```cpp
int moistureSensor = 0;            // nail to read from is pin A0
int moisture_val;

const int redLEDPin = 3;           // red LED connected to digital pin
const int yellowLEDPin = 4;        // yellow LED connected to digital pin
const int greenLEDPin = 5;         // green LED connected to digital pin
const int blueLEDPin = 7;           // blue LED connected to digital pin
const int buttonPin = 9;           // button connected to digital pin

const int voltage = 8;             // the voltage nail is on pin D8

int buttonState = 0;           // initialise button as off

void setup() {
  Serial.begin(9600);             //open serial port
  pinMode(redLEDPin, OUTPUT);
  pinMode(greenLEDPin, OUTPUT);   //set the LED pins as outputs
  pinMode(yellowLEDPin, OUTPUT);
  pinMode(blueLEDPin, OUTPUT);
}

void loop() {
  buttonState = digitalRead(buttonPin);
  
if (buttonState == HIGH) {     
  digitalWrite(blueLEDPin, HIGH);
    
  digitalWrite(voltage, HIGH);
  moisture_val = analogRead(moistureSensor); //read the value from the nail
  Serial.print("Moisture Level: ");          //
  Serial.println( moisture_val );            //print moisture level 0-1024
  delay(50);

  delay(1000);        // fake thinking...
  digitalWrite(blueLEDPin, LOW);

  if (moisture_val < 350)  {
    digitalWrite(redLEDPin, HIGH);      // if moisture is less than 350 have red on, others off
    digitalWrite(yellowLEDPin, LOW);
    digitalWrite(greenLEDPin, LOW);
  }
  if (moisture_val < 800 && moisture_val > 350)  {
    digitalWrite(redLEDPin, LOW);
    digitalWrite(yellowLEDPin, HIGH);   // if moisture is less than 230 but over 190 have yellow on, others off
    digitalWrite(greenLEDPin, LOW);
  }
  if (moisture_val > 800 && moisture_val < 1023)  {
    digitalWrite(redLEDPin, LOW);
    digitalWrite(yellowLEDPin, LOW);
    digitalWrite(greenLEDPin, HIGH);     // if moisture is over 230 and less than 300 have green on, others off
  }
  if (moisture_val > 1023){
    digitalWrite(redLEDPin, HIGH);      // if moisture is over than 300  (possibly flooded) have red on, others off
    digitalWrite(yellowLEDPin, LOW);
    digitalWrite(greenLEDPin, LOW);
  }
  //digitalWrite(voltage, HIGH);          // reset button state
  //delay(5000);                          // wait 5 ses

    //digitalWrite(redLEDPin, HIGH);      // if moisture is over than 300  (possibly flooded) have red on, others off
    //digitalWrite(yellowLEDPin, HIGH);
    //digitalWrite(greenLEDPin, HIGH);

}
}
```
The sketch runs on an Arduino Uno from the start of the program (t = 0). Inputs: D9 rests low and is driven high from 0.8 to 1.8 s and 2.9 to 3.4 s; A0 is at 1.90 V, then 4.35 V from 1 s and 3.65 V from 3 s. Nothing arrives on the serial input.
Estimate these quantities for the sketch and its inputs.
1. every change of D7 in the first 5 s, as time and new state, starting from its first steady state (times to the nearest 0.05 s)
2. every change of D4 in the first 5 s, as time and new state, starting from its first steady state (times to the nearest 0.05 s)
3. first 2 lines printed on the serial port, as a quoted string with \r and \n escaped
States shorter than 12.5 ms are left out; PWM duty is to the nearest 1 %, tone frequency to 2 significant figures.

0 s low; 0.8 s high; 1.85 s low; 2.9 s high; 3.95 s low
0 s low; 1.85 s high; 3.95 s low
"Moisture Level: 389\r\nMoisture Level: 890\r\n"
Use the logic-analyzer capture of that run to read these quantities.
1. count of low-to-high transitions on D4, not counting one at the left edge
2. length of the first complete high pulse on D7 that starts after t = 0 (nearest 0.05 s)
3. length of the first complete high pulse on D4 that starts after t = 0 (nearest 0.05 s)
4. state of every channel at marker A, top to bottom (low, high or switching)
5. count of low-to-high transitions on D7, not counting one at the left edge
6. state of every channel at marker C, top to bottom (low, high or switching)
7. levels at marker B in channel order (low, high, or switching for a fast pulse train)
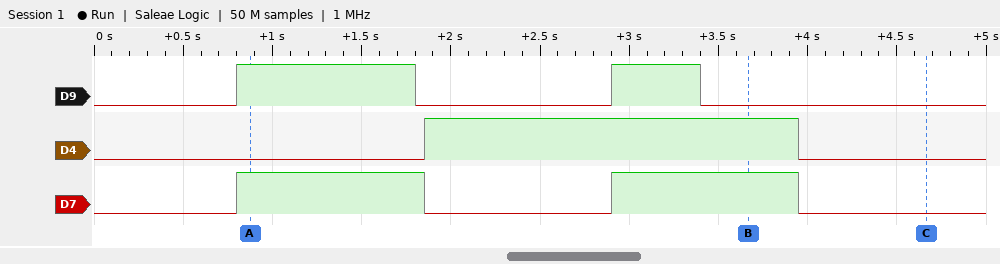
1
1.05 s
2.10 s
D9 high, D4 low, D7 high
2
D9 low, D4 low, D7 low
D9 low, D4 high, D7 high
